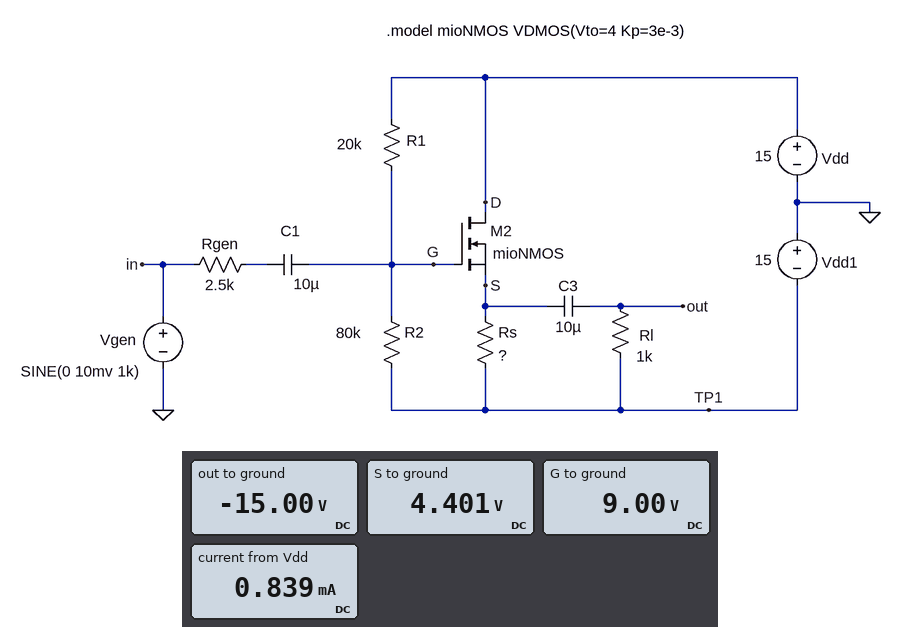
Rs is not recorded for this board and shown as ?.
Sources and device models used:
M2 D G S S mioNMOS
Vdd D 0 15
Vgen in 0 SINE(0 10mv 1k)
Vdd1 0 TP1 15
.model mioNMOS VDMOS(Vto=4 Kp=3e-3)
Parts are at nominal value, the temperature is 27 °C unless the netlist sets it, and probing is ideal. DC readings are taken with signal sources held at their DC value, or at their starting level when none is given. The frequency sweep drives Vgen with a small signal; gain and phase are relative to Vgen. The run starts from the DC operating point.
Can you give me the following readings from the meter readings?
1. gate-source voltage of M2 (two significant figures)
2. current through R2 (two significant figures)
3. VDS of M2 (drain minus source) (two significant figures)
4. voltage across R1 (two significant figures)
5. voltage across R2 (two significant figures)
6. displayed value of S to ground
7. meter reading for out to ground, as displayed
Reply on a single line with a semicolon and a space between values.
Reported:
4.6 V; 300 µA; 11 V; 6.0 V; 24 V; 4.401 V; -15.00 V
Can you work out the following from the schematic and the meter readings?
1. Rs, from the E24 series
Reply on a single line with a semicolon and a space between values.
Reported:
36 kΩ
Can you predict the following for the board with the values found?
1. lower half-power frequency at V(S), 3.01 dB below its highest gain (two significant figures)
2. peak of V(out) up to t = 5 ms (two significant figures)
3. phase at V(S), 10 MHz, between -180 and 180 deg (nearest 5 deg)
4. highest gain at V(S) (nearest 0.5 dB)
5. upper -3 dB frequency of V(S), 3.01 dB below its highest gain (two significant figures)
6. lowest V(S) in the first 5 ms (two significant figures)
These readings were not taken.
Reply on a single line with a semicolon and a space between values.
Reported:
770 mHz; -15 V; -85 deg; -2.0 dB; 47 Hz; 4.4 V
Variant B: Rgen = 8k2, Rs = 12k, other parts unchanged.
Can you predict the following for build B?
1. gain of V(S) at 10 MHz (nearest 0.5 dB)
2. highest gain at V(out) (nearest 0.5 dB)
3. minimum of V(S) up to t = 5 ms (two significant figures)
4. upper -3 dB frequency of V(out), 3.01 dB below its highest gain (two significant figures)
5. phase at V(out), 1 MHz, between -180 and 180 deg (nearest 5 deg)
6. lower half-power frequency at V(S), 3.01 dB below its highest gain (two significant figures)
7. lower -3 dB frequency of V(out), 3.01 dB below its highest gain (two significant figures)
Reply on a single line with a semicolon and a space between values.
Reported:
-43.5 dB; -6.0 dB; 4.0 V; 55 kHz; -65 deg; 620 mHz; 12 Hz
